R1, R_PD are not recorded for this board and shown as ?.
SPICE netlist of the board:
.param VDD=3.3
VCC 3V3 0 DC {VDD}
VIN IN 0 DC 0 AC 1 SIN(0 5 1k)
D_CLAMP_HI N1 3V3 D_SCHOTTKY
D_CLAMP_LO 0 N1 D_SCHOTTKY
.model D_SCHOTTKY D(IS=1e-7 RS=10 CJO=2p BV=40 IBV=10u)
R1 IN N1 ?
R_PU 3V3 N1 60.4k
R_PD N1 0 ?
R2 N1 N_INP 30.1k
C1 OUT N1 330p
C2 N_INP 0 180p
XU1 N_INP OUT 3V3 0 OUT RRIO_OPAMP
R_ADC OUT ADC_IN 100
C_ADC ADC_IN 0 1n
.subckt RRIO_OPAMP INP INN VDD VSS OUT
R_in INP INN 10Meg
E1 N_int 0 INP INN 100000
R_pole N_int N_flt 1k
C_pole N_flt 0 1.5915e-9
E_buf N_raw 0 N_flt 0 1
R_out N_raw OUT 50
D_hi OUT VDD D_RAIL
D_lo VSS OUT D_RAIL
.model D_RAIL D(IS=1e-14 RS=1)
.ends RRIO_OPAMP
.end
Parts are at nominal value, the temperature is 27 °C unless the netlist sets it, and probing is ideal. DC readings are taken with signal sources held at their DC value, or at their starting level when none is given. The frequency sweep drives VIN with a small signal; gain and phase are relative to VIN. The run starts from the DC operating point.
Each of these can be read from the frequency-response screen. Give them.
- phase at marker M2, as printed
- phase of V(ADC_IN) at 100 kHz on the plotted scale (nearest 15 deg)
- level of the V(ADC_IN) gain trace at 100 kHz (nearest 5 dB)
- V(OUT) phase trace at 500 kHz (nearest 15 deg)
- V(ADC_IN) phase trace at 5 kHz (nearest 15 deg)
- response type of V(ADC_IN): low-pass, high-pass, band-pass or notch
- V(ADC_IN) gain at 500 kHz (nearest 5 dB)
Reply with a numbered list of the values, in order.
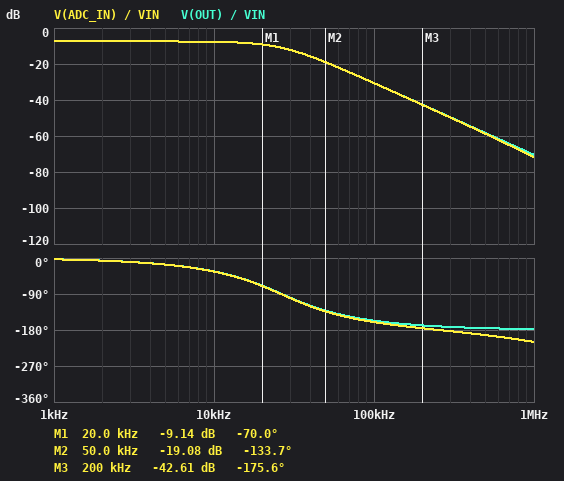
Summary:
1. -133.7 deg
2. -165 deg
3. -30 dB
4. -180 deg
5. -15 deg
6. low-pass
7. -60 dB
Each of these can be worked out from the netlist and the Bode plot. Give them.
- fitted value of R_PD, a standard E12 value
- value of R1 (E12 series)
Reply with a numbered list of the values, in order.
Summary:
1. 82 kΩ
2. 47 kΩ
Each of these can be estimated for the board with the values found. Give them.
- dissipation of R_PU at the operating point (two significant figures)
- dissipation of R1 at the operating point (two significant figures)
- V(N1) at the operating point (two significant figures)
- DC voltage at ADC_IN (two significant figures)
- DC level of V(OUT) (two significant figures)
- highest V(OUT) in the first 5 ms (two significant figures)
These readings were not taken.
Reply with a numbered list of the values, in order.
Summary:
1. 81 µW
2. 25 µW
3. 1.1 V
4. 1.1 V
5. 1.1 V
6. 3.2 V
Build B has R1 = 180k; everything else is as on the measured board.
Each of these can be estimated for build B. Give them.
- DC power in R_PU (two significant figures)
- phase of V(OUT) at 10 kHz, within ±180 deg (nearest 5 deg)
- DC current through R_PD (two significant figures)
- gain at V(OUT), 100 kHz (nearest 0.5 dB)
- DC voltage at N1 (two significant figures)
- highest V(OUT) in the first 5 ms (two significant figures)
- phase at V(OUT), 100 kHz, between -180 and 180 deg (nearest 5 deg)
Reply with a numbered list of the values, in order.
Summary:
1. 48 µW
2. -40 deg
3. 19 µA
4. -42.0 dB
5. 1.6 V
6. 2.4 V
7. -160 deg
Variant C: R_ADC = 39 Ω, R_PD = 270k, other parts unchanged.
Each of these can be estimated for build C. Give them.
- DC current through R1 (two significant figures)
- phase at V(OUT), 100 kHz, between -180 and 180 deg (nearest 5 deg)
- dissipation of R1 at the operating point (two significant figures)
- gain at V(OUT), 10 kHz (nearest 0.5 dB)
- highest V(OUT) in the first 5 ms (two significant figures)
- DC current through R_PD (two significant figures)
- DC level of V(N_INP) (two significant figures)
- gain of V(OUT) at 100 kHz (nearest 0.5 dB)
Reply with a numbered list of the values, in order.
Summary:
1. 28 µA
2. -160 deg
3. 37 µW
4. -6.0 dB
5. 3.4 V
6. 4.9 µA
7. 1.3 V
8. -30.5 dB
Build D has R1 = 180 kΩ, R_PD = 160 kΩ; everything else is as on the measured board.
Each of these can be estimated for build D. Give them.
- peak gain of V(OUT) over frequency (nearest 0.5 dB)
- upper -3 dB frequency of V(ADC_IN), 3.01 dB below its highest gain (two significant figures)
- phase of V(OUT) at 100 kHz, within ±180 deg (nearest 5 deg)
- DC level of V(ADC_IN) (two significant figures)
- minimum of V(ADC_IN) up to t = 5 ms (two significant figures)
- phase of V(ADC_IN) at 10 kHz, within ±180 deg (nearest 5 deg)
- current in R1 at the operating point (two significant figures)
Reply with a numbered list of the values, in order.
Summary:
1. -14.0 dB
2. 19 kHz
3. -165 deg
4. 1.9 V
5. 950 mV
6. -45 deg
7. 11 µA
